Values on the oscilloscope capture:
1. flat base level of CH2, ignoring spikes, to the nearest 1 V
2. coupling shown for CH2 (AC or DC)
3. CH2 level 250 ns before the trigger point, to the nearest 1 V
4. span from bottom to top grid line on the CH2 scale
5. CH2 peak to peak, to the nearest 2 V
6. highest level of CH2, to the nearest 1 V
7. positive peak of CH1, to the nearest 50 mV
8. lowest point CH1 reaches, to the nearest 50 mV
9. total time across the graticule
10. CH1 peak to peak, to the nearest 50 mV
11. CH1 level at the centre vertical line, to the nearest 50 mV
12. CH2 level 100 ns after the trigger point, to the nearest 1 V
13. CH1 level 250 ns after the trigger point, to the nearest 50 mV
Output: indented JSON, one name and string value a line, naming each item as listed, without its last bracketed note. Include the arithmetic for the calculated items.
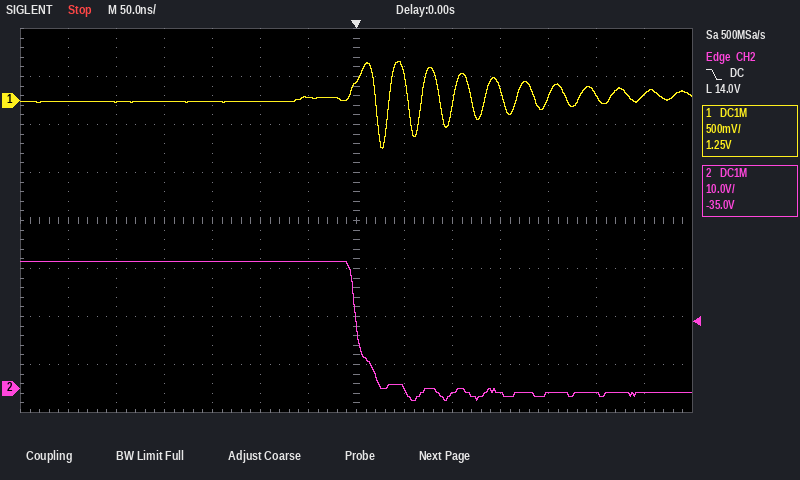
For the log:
{
  "flat base level of CH2, ignoring spikes, to the nearest 1 V": "-1 V",
  "coupling shown for CH2": "DC",
  "CH2 level 250 ns before the trigger point, to the nearest 1 V": "26 V",
  "span from bottom to top grid line on the CH2 scale": "80 V",
  "CH2 peak to peak, to the nearest 2 V": "28 V",
  "highest level of CH2, to the nearest 1 V": "26 V",
  "positive peak of CH1, to the nearest 50 mV": "400 mV",
  "lowest point CH1 reaches, to the nearest 50 mV": "-500 mV",
  "total time across the graticule": "700 ns",
  "CH1 peak to peak, to the nearest 50 mV": "400 mV − (-500 mV) = 900 mV",
  "CH1 level at the centre vertical line, to the nearest 50 mV": "200 mV",
  "CH2 level 100 ns after the trigger point, to the nearest 1 V": "-1 V",
  "CH1 level 250 ns after the trigger point, to the nearest 50 mV": "50 mV"
}
